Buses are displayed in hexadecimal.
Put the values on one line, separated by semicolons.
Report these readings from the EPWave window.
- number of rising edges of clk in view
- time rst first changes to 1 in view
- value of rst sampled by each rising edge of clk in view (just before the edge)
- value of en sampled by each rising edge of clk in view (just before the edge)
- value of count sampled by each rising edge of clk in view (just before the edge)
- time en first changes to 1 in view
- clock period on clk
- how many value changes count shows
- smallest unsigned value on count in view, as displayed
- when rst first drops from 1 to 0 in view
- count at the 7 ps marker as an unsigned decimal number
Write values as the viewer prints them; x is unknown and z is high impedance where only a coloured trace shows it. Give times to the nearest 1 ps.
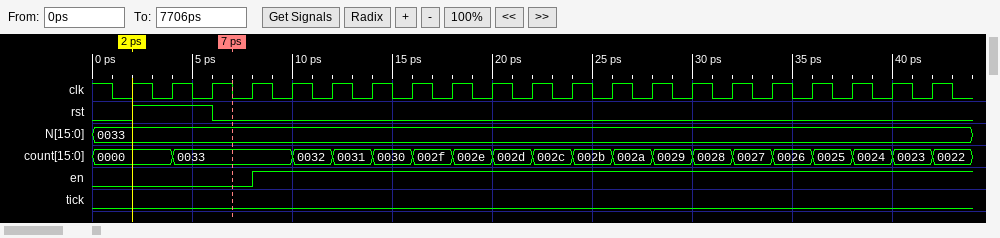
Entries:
21; 2 ps; 0 1 1 0 0 0 0 0 0 0 0 0 0 0 0 0 0 0 0 0 0; 0 0 0 0 1 1 1 1 1 1 1 1 1 1 1 1 1 1 1 1 1; 0000, 0000, 0033, 0033, 0033, 0032, 0031, 0030, 002f, 002e, 002d, 002c, 002b, 002a, 0029, 0028, 0027, 0026, 0025, 0024, 0023; 8 ps; 2 ps; 18; 0000; 6 ps; 51
